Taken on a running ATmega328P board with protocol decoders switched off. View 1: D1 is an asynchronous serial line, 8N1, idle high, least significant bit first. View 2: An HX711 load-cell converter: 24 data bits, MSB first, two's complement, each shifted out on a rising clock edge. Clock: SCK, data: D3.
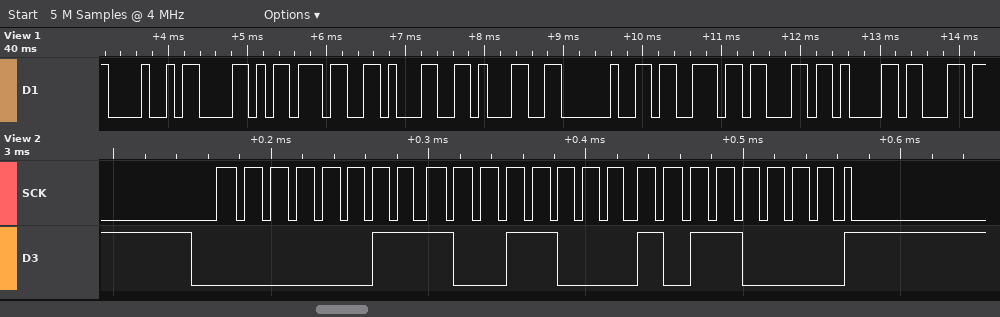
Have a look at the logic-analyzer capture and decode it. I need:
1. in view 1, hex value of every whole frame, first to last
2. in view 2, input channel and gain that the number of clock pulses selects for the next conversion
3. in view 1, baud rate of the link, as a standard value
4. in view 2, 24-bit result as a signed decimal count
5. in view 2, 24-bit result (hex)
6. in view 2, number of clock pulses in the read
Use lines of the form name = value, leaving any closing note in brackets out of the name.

in view 1, hex value of every whole frame, first to last = 48 58 37 31 31 20 73 63 61
in view 2, input channel and gain that the number of clock pulses selects for the next conversion = channel A, gain 128
in view 1, baud rate of the link, as a standard value = 9600 baud
in view 2, 24-bit result as a signed decimal count = 235696
in view 2, 24-bit result = 0x0398B0
in view 2, number of clock pulses in the read = 25
